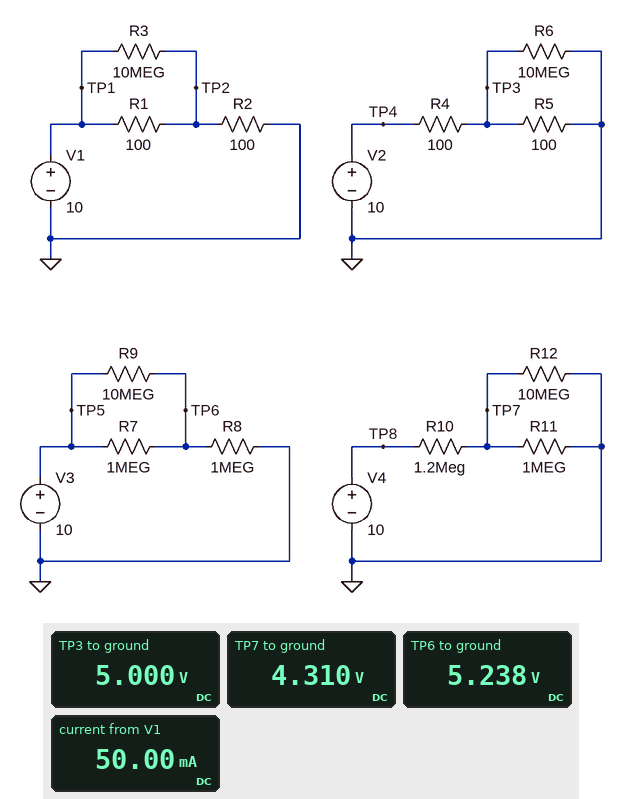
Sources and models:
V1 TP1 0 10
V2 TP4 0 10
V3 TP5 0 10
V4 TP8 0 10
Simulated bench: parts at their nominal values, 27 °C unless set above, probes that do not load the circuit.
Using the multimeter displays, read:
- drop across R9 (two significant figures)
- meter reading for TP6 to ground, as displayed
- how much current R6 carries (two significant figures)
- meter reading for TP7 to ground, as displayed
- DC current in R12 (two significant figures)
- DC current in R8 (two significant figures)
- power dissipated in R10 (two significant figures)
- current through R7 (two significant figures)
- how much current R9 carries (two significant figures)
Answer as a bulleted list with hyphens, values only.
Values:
- 4.8 V
- 5.238 V
- 500 nA
- 4.310 V
- 430 nA
- 5.2 µA
- 27 µW
- 4.8 µA
- 480 nA
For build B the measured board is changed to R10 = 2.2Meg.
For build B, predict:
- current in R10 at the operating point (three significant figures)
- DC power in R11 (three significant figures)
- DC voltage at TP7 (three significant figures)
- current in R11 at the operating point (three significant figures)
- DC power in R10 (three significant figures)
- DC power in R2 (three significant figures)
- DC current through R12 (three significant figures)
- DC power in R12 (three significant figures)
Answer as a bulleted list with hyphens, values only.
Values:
- 3.22 µA
- 8.55 µW
- 2.92 V
- 2.92 µA
- 22.8 µW
- 250 mW
- 292 nA
- 855 nW
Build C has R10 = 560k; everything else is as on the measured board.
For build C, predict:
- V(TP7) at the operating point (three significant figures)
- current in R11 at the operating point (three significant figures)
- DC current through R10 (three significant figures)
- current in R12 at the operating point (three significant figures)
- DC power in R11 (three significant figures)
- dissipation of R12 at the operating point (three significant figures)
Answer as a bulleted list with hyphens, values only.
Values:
- 6.19 V
- 6.19 µA
- 6.81 µA
- 619 nA
- 38.3 µW
- 3.83 µW
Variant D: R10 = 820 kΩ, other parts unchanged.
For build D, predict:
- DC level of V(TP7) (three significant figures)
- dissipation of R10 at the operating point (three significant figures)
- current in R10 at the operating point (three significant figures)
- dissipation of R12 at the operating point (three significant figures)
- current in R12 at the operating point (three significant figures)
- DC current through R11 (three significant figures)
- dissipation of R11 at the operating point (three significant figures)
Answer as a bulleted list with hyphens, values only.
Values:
- 5.26 V
- 27.4 µW
- 5.78 µA
- 2.76 µW
- 526 nA
- 5.26 µA
- 27.6 µW
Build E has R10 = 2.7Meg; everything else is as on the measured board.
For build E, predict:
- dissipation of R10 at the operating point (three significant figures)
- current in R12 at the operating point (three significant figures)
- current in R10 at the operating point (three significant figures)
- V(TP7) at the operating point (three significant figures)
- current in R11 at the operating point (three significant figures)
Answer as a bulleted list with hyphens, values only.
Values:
- 20.7 µW
- 252 nA
- 2.77 µA
- 2.52 V
- 2.52 µA
